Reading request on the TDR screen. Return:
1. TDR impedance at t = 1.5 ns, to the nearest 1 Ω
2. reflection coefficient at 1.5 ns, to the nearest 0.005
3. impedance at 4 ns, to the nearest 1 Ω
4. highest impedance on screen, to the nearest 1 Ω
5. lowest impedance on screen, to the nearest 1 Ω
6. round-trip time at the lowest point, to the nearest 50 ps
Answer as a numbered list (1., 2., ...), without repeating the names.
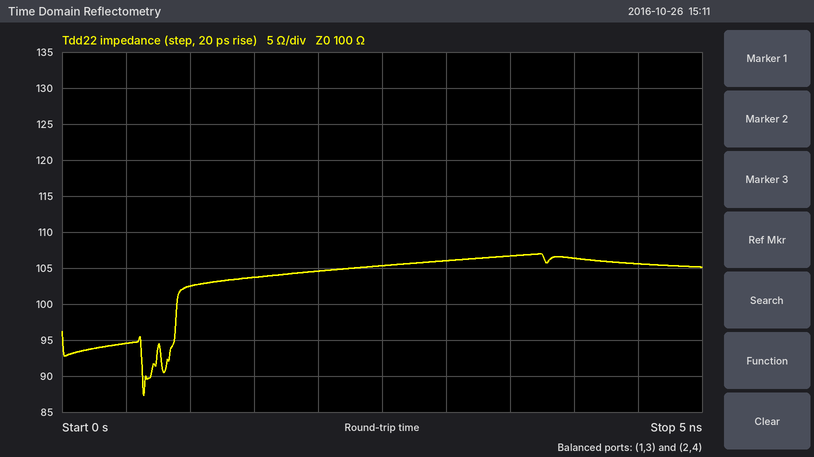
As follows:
1. 104 Ω
2. +0.020
3. 106 Ω
4. 107 Ω
5. 87 Ω
6. 650 ps
